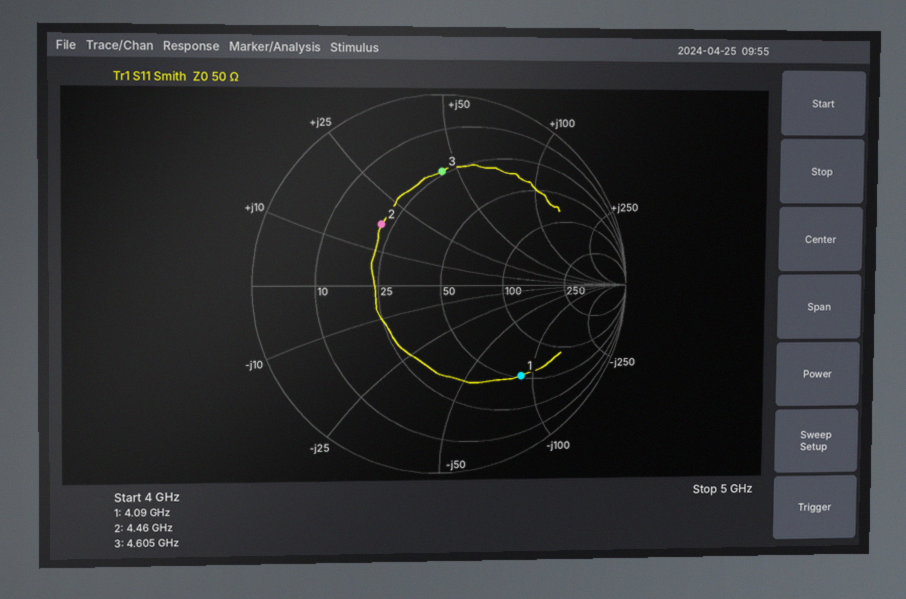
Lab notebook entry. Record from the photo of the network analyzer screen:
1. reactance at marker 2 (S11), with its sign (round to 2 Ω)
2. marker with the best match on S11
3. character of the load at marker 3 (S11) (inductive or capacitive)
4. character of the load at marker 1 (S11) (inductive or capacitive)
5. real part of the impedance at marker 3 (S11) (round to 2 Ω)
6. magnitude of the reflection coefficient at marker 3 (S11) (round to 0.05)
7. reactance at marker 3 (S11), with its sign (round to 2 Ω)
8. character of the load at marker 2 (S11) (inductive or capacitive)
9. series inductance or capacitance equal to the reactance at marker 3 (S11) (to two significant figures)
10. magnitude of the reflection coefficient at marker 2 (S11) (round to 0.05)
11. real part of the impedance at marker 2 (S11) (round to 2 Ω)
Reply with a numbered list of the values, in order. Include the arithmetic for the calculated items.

1. +18 Ω
2. marker 2
3. inductive
4. capacitive
5. 24 Ω
6. 0.60
7. +44 Ω
8. inductive
9. L = 44 Ω/(2π × 4.605 GHz) ≈ 1.5 nH
10. 0.45
11. 22 Ω
